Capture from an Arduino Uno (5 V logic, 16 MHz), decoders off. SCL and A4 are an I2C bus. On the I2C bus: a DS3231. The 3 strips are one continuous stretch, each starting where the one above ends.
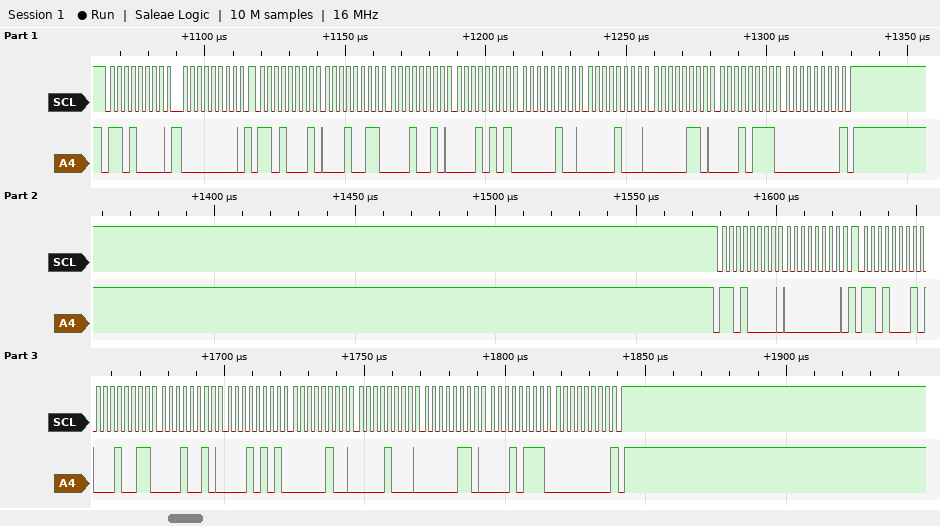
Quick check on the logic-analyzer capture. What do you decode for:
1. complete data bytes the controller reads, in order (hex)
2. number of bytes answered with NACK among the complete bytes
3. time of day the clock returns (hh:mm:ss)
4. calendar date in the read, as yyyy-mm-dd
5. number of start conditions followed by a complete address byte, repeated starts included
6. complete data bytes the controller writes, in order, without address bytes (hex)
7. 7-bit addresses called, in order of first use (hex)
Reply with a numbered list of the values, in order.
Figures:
1. 13 12 15 04 08 06 17 00 13 12 15 04 08 06 17 00
2. 2
3. 15:12:13
4. 2017-06-08
5. 4
6. 00 00
7. 0x68
